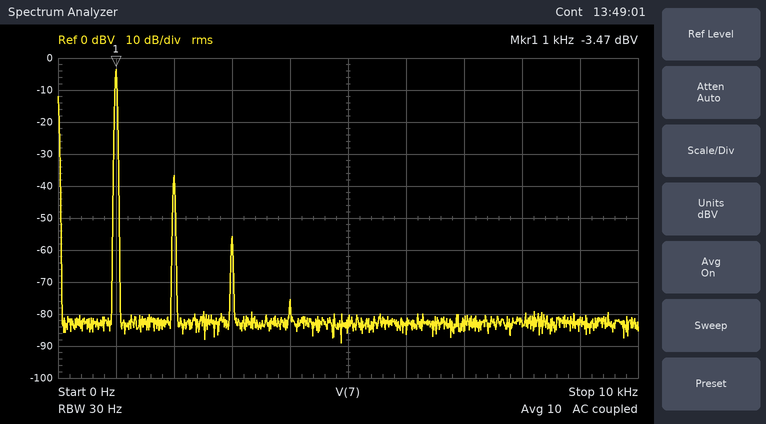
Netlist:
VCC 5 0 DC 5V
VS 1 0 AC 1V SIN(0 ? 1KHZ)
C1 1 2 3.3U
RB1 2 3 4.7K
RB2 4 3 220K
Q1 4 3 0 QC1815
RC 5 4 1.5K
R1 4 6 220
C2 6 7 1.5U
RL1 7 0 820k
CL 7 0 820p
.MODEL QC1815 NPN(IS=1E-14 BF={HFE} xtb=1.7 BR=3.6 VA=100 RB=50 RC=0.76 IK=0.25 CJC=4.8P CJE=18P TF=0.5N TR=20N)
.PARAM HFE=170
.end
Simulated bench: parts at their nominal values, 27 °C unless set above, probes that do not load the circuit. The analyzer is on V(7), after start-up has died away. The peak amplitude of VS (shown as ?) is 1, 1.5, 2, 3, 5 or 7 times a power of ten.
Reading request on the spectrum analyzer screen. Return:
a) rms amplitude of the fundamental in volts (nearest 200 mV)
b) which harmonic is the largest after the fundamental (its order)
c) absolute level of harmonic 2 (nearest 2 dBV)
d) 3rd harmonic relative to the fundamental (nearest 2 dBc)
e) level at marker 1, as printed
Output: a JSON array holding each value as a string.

["600 mV", "2", "-36 dBV", "-52 dBc", "-3.47 dBV"]
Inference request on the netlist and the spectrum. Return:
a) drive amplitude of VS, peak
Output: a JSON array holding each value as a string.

["50 mV"]
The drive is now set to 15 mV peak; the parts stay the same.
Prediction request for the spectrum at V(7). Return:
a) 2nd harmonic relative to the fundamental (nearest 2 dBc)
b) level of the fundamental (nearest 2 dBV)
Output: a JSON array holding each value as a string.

["-44 dBc", "-14 dBV"]
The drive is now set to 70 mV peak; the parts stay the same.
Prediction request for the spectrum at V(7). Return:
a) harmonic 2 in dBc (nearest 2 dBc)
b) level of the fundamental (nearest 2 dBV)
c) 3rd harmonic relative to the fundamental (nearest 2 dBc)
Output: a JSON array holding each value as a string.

["-30 dBc", "0 dBV", "-46 dBc"]
